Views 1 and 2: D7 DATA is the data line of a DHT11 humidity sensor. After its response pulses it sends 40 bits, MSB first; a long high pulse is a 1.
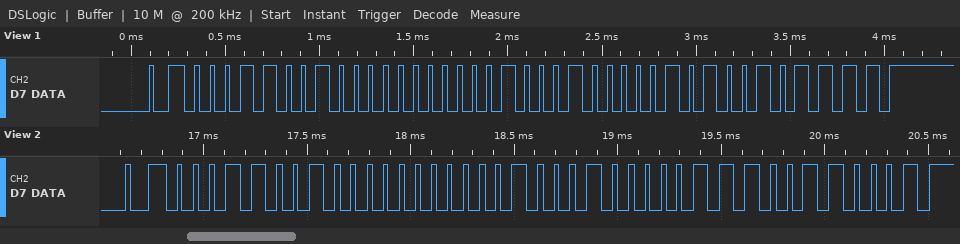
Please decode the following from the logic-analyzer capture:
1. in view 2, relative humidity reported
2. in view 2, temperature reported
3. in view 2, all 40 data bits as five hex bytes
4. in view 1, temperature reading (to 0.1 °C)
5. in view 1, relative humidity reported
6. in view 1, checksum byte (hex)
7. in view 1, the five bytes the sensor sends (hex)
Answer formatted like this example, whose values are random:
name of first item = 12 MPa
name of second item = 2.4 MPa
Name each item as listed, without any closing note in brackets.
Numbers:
in view 2, relative humidity reported = 25 %
in view 2, temperature reported = 17.7 °C
in view 2, all 40 data bits as five hex bytes = 19 00 11 07 31
in view 1, temperature reading = 17.5 °C
in view 1, relative humidity reported = 25 %
in view 1, checksum byte = 0x2F
in view 1, the five bytes the sensor sends = 19 00 11 05 2F
